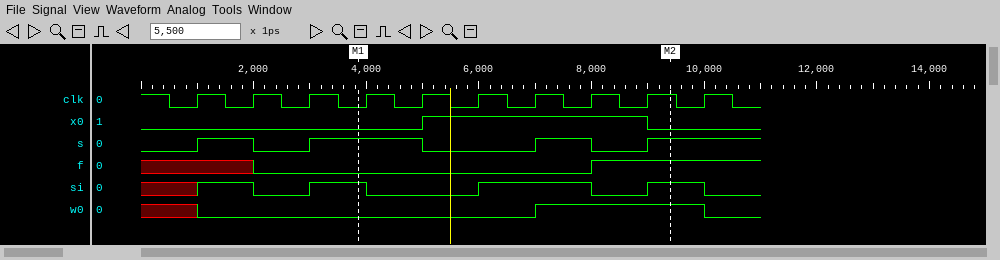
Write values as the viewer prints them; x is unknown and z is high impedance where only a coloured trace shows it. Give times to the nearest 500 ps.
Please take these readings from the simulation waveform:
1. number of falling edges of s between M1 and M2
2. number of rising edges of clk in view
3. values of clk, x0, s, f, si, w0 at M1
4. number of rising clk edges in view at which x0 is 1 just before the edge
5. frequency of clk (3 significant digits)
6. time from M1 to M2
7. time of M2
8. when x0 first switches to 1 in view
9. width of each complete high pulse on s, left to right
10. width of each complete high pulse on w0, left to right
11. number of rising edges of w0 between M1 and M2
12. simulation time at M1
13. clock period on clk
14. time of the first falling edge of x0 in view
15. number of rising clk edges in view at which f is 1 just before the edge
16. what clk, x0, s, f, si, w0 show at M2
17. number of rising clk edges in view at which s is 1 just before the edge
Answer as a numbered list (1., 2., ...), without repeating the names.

1. 2
2. 10
3. clk=0, x0=0, s=1, f=0, si=1, w0=0
4. 4
5. 1.00 GHz
6. 5500 ps
7. 9500 ps
8. 5000 ps
9. 1000 ps, 2000 ps, 1000 ps
10. 3000 ps
11. 1
12. 4000 ps
13. 1000 ps
14. 9000 ps
15. 2
16. clk=1, x0=0, s=1, f=1, si=1, w0=1
17. 5
